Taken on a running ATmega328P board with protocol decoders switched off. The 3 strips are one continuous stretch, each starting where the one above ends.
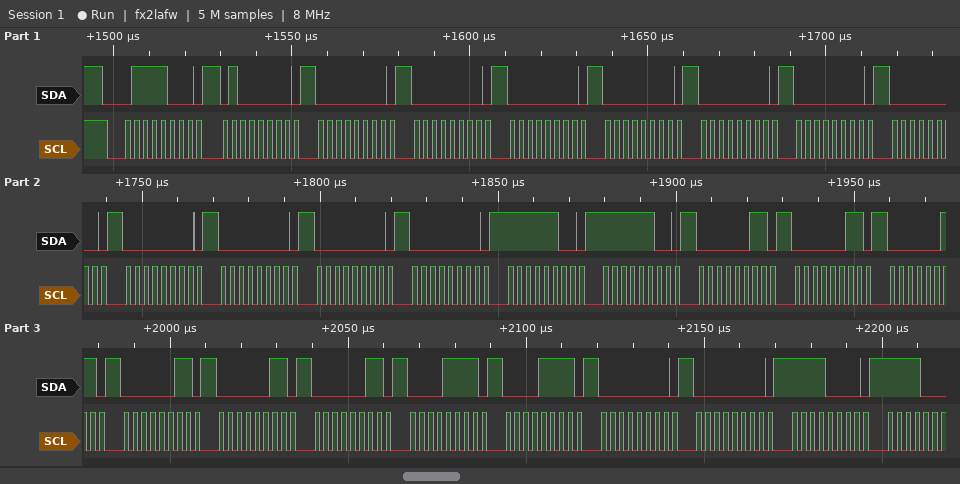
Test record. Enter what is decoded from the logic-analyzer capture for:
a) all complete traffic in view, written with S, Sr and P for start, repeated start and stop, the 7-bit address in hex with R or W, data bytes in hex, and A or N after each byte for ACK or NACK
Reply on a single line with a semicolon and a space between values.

S 3CW A 40 A 00 A 00 A 00 A 00 A 00 A 00 A 00 A 00 A 00 A 00 A 00 A FC A FC A 03 A 03 A 03 A 03 A 03 A 03 A 0F A 0F A 00 A 00 A F0 A
